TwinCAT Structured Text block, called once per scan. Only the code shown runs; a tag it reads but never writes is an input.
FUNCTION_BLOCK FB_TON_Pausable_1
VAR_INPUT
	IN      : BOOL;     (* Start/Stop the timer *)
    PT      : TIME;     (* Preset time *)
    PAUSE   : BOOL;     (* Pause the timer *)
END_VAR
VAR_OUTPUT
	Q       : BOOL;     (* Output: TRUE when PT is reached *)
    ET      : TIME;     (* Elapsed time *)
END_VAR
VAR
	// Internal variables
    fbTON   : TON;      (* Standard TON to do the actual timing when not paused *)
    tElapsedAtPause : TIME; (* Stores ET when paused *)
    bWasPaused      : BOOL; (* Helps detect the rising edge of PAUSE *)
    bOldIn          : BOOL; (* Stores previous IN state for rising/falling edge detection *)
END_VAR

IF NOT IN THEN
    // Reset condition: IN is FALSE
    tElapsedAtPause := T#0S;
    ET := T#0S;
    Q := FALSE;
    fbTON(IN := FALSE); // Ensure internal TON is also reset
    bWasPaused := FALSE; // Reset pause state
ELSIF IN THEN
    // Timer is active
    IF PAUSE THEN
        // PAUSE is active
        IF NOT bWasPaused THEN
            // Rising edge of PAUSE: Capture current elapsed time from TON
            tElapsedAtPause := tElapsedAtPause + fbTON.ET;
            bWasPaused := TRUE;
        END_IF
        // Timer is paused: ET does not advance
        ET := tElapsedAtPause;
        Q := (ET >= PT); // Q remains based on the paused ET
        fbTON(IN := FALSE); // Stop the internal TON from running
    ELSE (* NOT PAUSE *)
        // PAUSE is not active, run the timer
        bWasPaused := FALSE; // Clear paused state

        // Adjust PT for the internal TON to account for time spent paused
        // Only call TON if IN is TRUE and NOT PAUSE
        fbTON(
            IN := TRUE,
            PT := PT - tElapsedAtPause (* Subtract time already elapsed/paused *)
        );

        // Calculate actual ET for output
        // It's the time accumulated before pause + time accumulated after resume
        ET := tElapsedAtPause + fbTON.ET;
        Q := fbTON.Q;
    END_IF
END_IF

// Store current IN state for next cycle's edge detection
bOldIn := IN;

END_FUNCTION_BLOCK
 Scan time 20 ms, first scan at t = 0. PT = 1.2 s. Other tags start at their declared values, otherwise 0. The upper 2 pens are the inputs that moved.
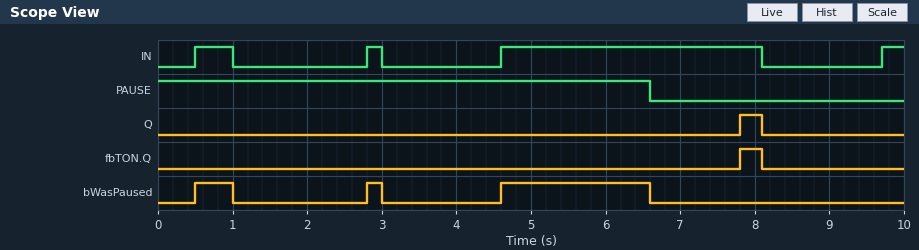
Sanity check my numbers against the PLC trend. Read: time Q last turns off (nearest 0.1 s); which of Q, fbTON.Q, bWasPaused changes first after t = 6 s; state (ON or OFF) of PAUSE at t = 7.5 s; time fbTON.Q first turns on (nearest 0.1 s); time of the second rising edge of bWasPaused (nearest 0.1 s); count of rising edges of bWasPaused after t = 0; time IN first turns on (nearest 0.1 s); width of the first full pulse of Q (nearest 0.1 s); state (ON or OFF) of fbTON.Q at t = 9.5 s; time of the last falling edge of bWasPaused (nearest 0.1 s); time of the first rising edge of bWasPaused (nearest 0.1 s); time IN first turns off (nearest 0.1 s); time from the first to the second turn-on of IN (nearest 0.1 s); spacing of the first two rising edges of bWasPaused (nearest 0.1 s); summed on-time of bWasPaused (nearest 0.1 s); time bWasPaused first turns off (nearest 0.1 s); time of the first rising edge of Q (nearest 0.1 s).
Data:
8.1 s
bWasPaused
OFF
7.8 s
2.8 s
3
0.5 s
0.3 s
OFF
6.6 s
0.5 s
1.0 s
2.3 s
2.3 s
2.7 s
1.0 s
7.8 s
